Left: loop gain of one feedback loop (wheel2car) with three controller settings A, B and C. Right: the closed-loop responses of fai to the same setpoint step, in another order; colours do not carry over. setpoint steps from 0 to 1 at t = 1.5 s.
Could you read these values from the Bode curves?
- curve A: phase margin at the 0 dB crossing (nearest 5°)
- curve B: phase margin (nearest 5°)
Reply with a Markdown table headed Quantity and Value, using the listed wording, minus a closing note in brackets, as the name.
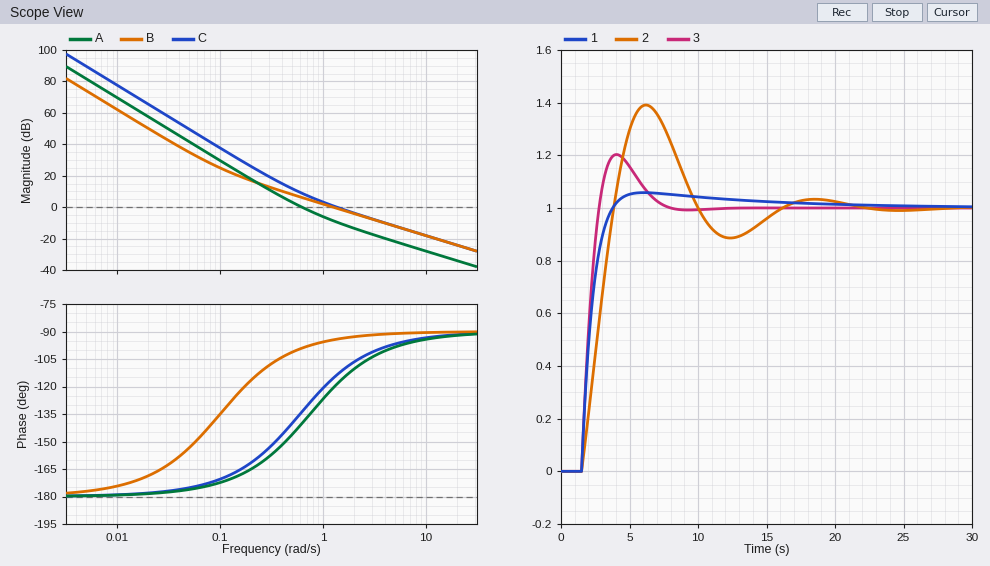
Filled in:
| Quantity | Value |
|---|---|
| curve A: phase margin at the 0 dB crossing | 40° |
| curve B: phase margin | 85° |
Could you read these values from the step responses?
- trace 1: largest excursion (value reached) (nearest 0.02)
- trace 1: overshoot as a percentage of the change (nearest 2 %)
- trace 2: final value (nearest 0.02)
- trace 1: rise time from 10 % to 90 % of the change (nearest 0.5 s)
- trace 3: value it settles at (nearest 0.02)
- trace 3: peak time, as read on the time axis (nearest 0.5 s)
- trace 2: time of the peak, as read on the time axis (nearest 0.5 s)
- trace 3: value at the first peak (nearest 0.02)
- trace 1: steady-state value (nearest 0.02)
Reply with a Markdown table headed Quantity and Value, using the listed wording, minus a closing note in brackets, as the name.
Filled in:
| Quantity | Value |
|---|---|
| trace 1: largest excursion (value reached) | 1.06 |
| trace 1: overshoot as a percentage of the change | 6 % |
| trace 2: final value | 1.00 |
| trace 1: rise time from 10 % to 90 % of the change | 1.5 s |
| trace 3: value it settles at | 1.00 |
| trace 3: peak time, as read on the time axis | 4.0 s |
| trace 2: time of the peak, as read on the time axis | 6.0 s |
| trace 3: value at the first peak | 1.20 |
| trace 1: steady-state value | 1.00 |
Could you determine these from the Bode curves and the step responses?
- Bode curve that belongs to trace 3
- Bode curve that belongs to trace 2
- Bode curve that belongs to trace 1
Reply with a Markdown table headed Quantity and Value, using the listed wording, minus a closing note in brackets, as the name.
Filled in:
| Quantity | Value |
|---|---|
| Bode curve that belongs to trace 3 | C |
| Bode curve that belongs to trace 2 | A |
| Bode curve that belongs to trace 1 | B |
